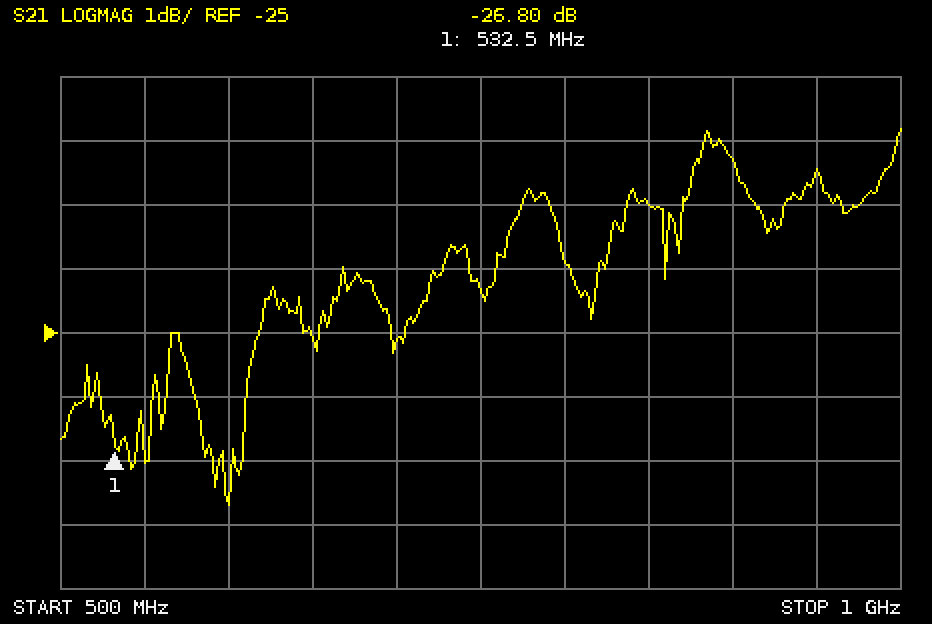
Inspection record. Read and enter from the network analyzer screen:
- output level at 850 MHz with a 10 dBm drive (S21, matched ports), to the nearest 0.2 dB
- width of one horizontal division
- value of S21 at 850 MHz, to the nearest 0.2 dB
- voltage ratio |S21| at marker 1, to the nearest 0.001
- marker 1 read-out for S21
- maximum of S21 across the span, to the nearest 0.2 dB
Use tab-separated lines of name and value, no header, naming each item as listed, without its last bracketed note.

output level at 850 MHz with a 10 dBm drive (S21, matched ports), to the nearest 0.2 dB	-13.0 dBm
width of one horizontal division	50 MHz
value of S21 at 850 MHz, to the nearest 0.2 dB	-23.0 dB
voltage ratio |S21| at marker 1, to the nearest 0.001	0.046
marker 1 read-out for S21	-26.80 dB
maximum of S21 across the span, to the nearest 0.2 dB	-21.8 dB
